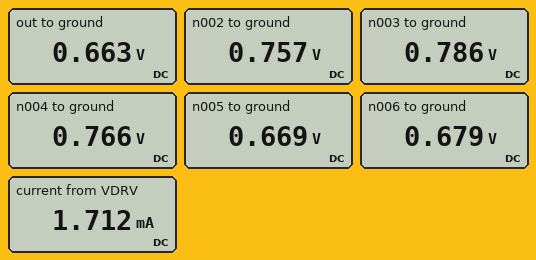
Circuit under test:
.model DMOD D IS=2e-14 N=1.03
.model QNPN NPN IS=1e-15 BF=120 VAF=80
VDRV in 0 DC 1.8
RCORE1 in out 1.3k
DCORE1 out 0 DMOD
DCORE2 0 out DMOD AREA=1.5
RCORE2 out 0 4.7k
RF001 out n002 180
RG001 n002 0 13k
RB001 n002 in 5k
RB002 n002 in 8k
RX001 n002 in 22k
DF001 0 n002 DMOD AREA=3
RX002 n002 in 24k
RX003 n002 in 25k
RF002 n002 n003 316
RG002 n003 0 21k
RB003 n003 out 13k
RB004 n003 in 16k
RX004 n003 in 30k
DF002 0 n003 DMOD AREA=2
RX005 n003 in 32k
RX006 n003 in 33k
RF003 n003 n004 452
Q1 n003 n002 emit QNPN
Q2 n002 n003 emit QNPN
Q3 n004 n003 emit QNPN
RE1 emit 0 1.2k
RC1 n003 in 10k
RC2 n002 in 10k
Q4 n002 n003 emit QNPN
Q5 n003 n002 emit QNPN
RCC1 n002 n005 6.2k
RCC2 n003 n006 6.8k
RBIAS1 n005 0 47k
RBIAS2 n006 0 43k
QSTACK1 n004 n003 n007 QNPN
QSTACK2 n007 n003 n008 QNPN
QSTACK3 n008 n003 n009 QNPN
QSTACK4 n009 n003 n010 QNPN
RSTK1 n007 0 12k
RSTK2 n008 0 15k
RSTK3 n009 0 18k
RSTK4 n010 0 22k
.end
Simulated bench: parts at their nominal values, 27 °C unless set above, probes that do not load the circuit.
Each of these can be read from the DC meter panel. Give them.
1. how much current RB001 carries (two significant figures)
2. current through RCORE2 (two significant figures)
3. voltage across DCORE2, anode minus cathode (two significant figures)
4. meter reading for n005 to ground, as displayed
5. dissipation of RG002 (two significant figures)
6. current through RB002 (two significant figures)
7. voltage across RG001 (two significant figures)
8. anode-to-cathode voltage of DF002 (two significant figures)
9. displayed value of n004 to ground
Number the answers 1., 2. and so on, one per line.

1. 210 µA
2. 140 µA
3. -660 mV
4. 0.669 V
5. 29 µW
6. 130 µA
7. 760 mV
8. -790 mV
9. 0.766 V
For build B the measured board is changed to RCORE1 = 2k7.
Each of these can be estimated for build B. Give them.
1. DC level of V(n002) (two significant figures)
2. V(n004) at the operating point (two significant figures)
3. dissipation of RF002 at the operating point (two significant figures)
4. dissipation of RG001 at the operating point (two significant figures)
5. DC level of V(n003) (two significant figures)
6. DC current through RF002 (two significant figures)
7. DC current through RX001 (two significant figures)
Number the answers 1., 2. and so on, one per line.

1. 750 mV
2. 760 mV
3. 3.1 µW
4. 43 µW
5. 780 mV
6. 99 µA
7. 48 µA
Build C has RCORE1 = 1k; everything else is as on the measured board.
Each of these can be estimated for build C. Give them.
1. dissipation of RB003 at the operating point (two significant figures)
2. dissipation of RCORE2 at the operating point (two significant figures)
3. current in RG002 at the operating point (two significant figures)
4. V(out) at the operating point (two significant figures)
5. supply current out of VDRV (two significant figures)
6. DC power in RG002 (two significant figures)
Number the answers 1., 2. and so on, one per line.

1. 1.1 µW
2. 95 µW
3. 38 µA
4. 670 mV
5. 2.0 mA
6. 30 µW
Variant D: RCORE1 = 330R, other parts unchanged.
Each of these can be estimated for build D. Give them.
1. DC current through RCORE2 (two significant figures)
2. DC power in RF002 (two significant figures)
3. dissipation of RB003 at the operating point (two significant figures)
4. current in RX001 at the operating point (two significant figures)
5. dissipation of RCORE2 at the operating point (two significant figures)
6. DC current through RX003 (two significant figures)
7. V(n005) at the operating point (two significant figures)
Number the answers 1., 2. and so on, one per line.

1. 150 µA
2. 1.8 µW
3. 960 nW
4. 46 µA
5. 100 µW
6. 41 µA
7. 690 mV
